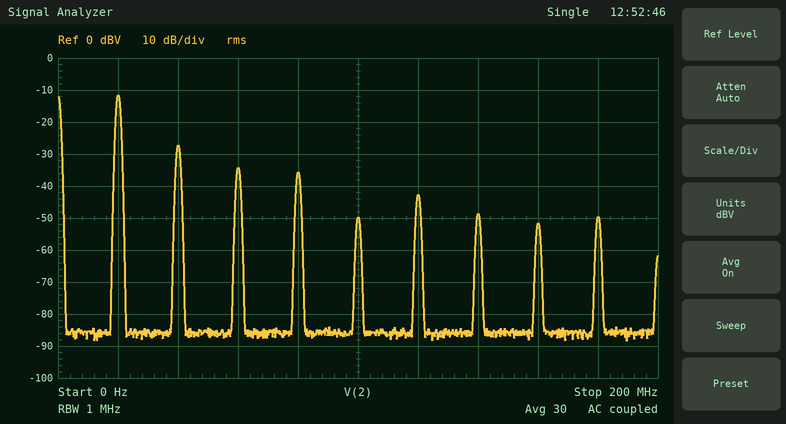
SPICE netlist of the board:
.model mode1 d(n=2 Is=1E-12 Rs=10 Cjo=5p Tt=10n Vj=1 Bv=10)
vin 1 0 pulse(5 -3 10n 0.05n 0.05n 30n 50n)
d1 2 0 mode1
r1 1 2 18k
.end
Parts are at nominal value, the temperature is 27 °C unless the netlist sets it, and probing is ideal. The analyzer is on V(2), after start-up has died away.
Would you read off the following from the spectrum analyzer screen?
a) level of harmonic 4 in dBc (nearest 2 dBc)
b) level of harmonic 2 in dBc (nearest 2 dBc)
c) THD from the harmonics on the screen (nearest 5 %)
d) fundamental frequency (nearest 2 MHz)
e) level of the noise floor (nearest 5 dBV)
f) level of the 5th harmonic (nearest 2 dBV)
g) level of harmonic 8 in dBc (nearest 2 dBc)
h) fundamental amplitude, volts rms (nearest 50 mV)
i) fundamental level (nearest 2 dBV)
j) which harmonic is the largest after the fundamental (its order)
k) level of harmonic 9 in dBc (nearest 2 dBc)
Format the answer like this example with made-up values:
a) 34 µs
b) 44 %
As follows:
a) -24 dBc
b) -16 dBc
c) 20 %
d) 20 MHz
e) -85 dBV
f) -50 dBV
g) -40 dBc
h) 250 mV
i) -12 dBV
j) 2
k) -38 dBc
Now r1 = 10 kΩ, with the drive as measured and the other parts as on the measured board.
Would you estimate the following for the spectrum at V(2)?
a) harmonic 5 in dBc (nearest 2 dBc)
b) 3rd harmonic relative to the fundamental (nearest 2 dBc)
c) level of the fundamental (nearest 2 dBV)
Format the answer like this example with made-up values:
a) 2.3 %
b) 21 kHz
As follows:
a) -34 dBc
b) -22 dBc
c) -6 dBV
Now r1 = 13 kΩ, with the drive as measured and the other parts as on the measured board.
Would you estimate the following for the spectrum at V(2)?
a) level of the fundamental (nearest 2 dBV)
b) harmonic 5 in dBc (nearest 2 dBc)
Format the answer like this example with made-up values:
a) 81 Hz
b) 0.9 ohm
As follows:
a) -8 dBV
b) -36 dBc
